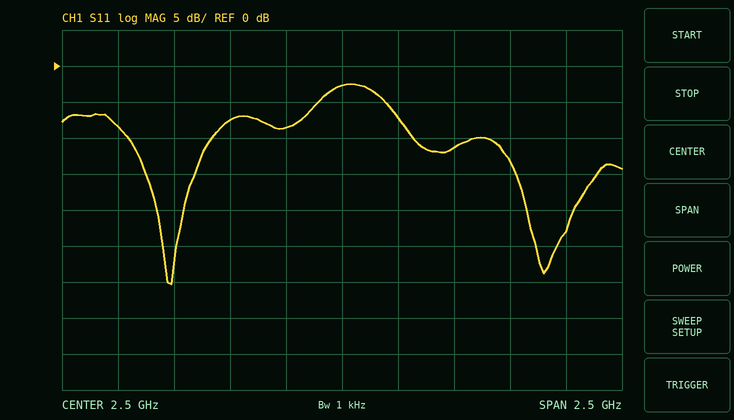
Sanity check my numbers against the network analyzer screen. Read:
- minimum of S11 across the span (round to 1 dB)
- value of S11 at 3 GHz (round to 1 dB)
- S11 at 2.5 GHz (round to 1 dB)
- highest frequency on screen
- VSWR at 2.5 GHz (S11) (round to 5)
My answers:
-30 dB
-11 dB
-3 dB
3.75 GHz
5
